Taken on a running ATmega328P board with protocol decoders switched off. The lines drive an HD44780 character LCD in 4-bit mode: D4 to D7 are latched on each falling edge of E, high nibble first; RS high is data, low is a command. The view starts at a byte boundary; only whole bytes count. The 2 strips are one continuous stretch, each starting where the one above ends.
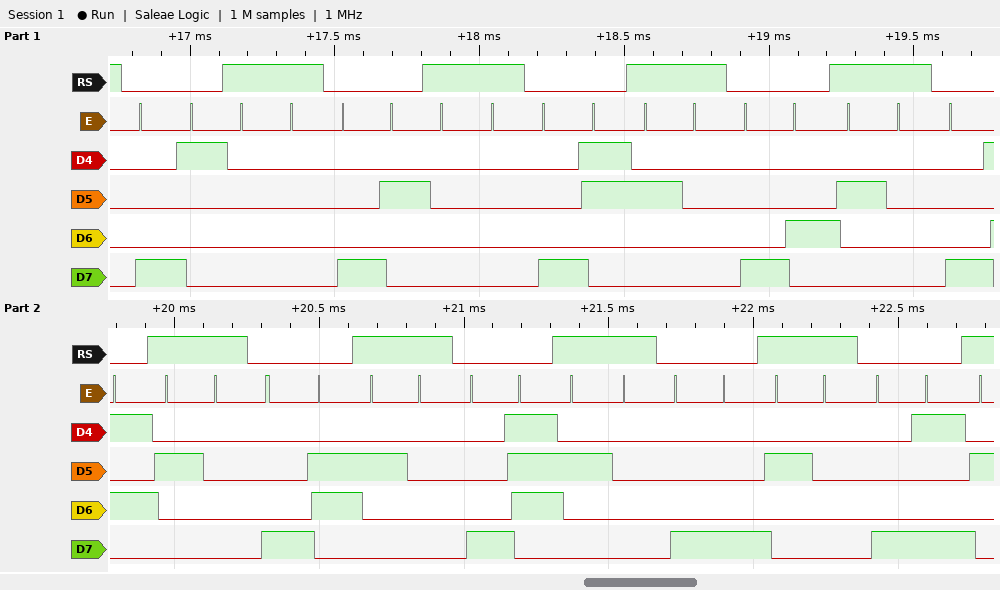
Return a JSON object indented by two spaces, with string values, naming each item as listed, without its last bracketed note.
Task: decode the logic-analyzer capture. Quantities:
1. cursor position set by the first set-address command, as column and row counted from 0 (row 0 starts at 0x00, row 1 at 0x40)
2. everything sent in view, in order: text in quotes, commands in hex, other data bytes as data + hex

{
  "cursor position set by the first set-address command, as column and row counted from 0": "column 1, row 0",
  "everything sent in view, in order: text in quotes, commands in hex, other data bytes as data + hex": "0x81 data 00 0x82 data 00 0x83 \" \" 0x84 \" \" 0x85 \" \" 0x86 \" \" 0x87 \" \" 0x88 \" \" 0x89"
}
